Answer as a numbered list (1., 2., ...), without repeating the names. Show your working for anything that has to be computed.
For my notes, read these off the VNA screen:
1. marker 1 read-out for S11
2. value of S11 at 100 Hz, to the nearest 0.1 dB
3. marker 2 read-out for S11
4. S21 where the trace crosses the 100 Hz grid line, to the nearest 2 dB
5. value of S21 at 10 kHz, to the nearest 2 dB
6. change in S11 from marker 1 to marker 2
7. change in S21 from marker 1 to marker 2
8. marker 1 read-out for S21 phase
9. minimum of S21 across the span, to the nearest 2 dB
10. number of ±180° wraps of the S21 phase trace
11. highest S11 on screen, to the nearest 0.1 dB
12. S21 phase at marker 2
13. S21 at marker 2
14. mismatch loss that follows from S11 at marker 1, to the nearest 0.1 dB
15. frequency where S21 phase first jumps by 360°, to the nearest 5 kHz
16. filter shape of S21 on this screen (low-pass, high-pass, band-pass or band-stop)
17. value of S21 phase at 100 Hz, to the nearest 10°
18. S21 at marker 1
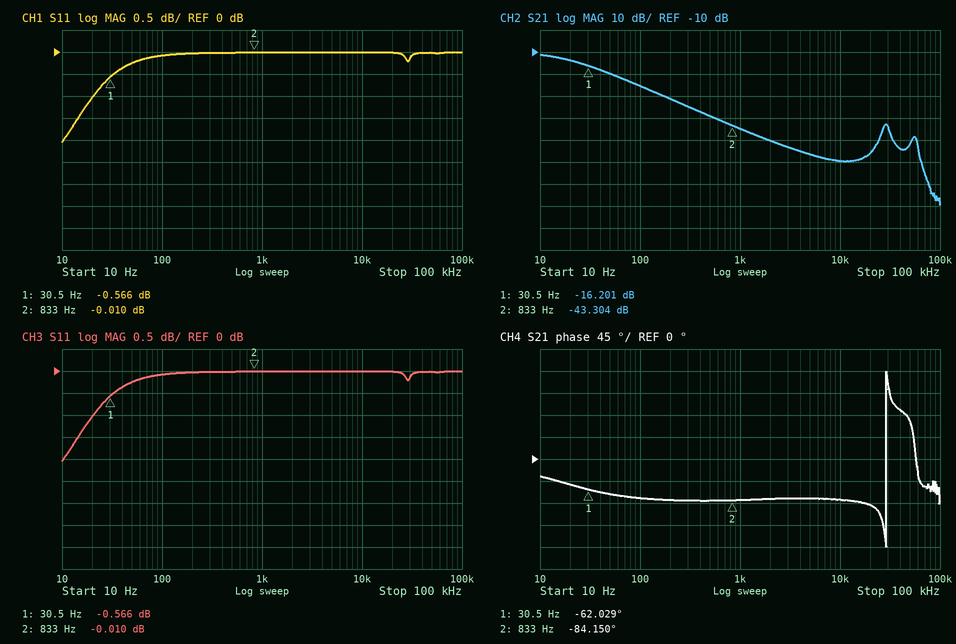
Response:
1. -0.566 dB
2. -0.1 dB
3. -0.010 dB
4. -26 dB
5. -60 dB
6. -0.01 − (-0.566) = 0.556 dB
7. -43.304 − (-16.201) = -27.103 dB
8. -62.029°
9. -80 dB
10. 1
11. 0.0 dB
12. -84.150°
13. -43.304 dB
14. −10 log10(1 − 10^(-0.566/10)) ≈ 9.1 dB
15. 30 kHz
16. low-pass
17. -80°
18. -16.201 dB
